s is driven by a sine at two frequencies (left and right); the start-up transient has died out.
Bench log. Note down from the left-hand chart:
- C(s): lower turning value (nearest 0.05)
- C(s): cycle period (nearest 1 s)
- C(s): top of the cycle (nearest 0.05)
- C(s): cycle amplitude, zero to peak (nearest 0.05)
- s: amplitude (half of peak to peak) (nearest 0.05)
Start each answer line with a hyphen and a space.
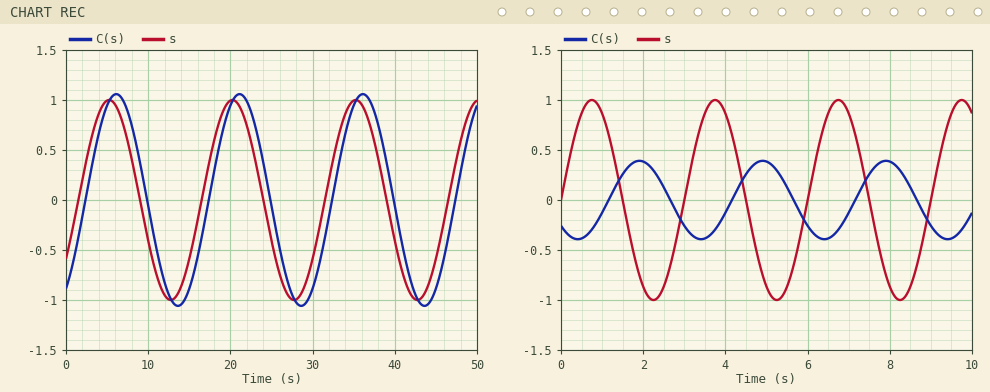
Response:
- -1.05
- 15 s
- 1.05
- 1.05
- 1.00
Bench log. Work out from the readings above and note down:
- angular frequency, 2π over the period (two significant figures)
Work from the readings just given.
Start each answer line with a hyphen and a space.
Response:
- 0.42 rad/s
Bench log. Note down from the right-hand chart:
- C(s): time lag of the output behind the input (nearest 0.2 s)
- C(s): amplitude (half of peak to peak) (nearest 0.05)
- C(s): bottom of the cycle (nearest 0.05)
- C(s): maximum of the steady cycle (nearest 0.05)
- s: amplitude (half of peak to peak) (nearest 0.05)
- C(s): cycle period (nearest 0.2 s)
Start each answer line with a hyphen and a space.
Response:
- 1.2 s
- 0.40
- -0.40
- 0.40
- 1.00
- 3.0 s
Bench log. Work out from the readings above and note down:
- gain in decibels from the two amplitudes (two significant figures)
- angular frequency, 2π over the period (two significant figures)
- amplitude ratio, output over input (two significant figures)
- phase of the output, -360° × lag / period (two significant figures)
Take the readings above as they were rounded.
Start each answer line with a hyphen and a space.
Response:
- -8.0 dB
- 2.1 rad/s
- 0.40
- -140°
